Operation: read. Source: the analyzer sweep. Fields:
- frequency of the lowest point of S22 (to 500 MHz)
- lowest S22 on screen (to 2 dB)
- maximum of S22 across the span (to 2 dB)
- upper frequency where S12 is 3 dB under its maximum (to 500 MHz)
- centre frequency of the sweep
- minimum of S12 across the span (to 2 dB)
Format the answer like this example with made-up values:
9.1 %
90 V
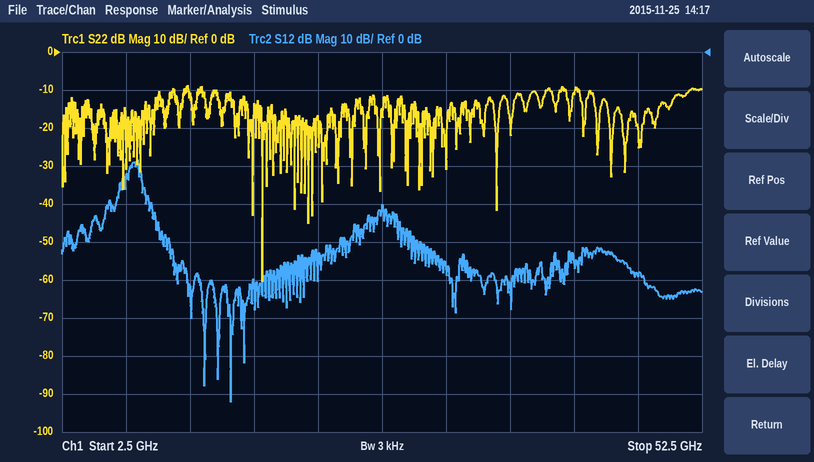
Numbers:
18.0 GHz
-60 dB
-8 dB
8.5 GHz
27.5 GHz
-92 dB
